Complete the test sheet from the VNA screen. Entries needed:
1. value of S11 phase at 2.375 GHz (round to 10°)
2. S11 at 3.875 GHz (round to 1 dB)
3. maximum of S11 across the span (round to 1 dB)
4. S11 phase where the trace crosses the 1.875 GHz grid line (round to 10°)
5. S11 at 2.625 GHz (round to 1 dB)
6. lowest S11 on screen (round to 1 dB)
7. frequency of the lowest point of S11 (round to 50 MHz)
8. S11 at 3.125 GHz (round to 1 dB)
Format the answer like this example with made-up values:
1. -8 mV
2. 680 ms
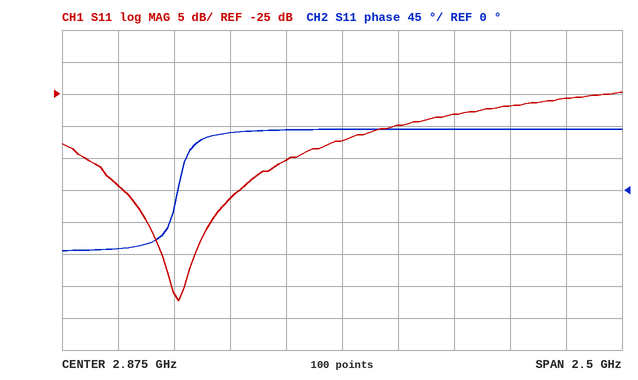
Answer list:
1. 80°
2. -26 dB
3. -25 dB
4. -80°
5. -35 dB
6. -57 dB
7. 2.15 GHz
8. -30 dB
